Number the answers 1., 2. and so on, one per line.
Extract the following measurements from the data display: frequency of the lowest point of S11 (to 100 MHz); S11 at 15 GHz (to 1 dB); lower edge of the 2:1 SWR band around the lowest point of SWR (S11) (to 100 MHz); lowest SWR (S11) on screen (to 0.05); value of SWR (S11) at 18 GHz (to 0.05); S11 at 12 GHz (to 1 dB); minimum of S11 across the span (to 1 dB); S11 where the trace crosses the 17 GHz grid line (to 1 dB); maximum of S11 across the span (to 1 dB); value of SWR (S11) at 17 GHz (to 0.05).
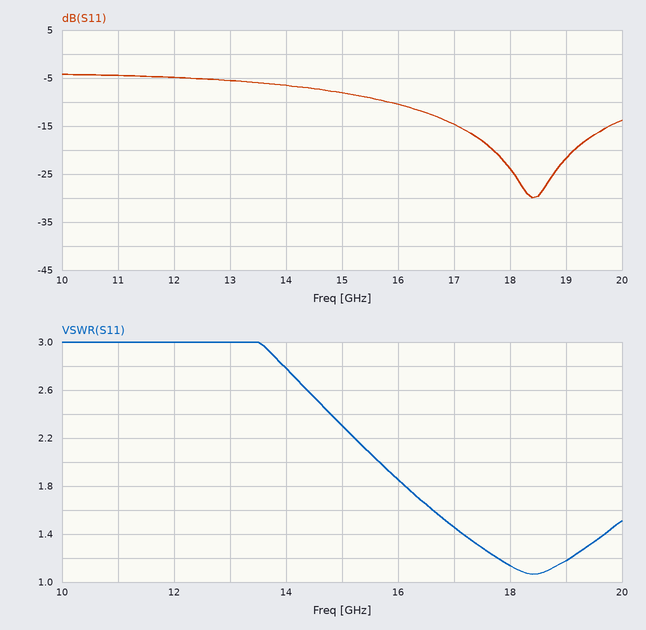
1. 18.4 GHz
2. -8 dB
3. 15.7 GHz
4. 1.05
5. 1.15
6. -5 dB
7. -30 dB
8. -15 dB
9. -4 dB
10. 1.45
